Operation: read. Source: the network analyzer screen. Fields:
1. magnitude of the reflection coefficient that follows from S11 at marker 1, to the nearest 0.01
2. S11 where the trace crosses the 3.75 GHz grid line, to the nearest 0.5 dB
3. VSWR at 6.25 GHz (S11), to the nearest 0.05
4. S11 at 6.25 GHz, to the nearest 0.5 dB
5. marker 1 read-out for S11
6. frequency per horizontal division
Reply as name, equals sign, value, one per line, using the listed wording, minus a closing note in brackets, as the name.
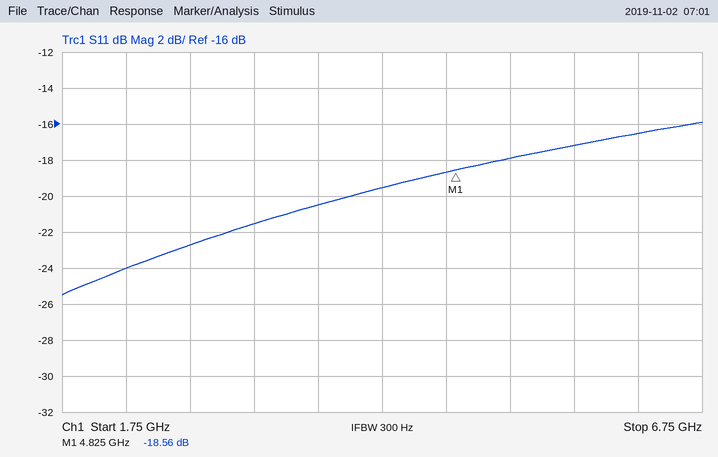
magnitude of the reflection coefficient that follows from S11 at marker 1, to the nearest 0.01 = 0.12
S11 where the trace crosses the 3.75 GHz grid line, to the nearest 0.5 dB = -20.5 dB
VSWR at 6.25 GHz (S11), to the nearest 0.05 = 1.35
S11 at 6.25 GHz, to the nearest 0.5 dB = -16.5 dB
marker 1 read-out for S11 = -18.56 dB
frequency per horizontal division = 500 MHz
